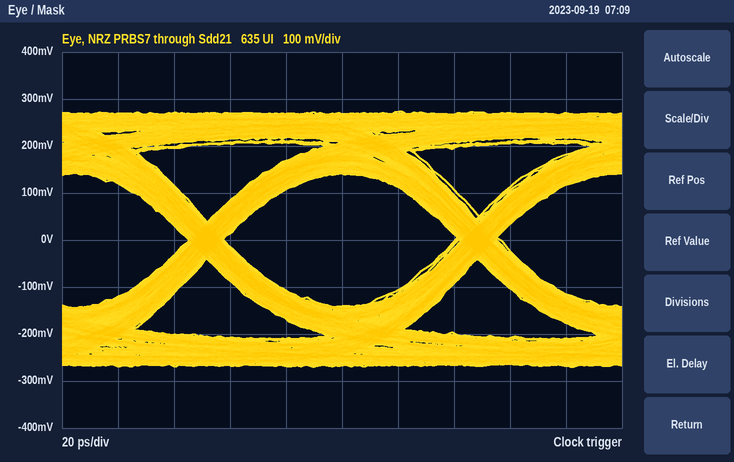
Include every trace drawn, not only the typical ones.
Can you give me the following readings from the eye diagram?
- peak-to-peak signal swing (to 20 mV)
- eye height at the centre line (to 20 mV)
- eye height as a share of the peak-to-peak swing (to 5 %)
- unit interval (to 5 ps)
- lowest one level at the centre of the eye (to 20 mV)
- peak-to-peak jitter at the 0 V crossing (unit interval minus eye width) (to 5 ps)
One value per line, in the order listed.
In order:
540 mV
280 mV
50 %
95 ps
140 mV
15 ps
